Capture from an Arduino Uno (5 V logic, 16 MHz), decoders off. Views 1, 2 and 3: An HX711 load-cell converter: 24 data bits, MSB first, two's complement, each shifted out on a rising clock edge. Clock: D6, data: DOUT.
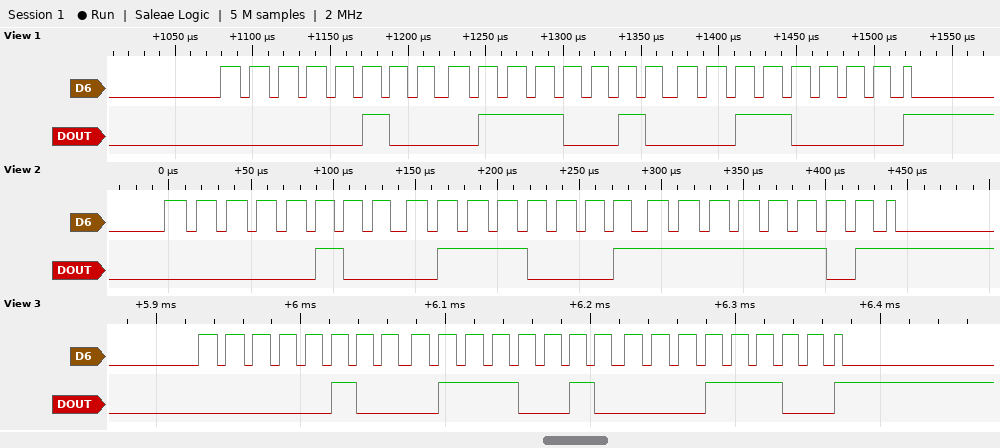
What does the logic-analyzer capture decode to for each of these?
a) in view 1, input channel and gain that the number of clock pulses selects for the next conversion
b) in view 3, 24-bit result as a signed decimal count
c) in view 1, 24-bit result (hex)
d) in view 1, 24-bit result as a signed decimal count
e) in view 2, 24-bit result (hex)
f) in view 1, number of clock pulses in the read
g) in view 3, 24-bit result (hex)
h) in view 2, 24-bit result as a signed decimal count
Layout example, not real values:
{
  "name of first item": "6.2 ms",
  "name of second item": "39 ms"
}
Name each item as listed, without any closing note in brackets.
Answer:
{
  "in view 1, input channel and gain that the number of clock pulses selects for the next conversion": "channel A, gain 128",
  "in view 3, 24-bit result as a signed decimal count": "291356",
  "in view 1, 24-bit result": "0x047230",
  "in view 1, 24-bit result as a signed decimal count": "291376",
  "in view 2, 24-bit result": "0x0471FD",
  "in view 1, number of clock pulses in the read": "25",
  "in view 3, 24-bit result": "0x04721C",
  "in view 2, 24-bit result as a signed decimal count": "291325"
}
